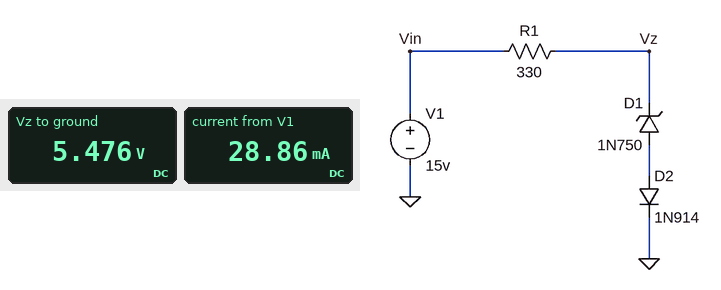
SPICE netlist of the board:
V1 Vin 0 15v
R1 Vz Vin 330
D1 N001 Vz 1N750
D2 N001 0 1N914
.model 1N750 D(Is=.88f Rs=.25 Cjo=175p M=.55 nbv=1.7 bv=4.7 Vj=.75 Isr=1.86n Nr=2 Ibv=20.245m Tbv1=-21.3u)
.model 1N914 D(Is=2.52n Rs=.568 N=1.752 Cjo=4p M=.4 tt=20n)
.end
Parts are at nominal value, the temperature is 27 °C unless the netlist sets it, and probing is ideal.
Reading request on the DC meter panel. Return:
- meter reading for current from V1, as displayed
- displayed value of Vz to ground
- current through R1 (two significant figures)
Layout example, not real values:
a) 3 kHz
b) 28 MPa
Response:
a) 28.86 mA
b) 5.476 V
c) 29 mA
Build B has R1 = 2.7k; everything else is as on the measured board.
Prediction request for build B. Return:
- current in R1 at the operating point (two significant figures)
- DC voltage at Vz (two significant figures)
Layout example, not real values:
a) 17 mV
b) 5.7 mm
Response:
a) 3.6 mA
b) 5.3 V
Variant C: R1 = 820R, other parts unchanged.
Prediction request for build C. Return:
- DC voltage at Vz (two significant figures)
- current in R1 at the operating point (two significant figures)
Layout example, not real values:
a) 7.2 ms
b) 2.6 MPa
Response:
a) 5.4 V
b) 12 mA
